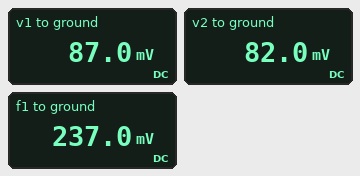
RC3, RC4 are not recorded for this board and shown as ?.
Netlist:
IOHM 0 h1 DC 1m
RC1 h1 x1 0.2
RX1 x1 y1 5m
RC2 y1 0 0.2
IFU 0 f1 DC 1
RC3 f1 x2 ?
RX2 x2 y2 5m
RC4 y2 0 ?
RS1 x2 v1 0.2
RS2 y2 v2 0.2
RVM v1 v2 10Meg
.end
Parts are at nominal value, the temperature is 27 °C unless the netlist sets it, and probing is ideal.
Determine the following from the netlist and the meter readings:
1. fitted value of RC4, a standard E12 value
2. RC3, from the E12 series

0.082 Ω
0.15 Ω
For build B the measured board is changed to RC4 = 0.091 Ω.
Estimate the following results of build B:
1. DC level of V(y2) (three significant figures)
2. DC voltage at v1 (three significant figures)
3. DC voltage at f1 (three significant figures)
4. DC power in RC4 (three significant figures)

91.0 mV
96.0 mV
246 mV
91.0 mW
